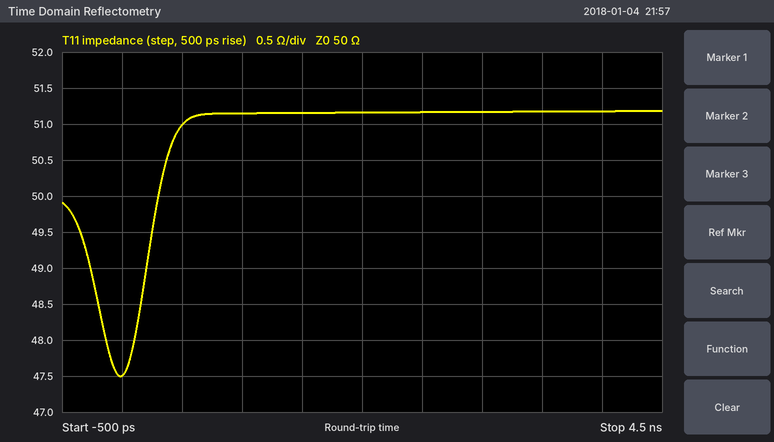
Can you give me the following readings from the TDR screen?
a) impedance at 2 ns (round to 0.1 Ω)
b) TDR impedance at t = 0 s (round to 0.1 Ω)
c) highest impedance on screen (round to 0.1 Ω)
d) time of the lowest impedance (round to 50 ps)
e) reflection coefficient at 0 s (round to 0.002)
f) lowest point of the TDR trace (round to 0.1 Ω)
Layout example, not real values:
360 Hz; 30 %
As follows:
51.2 Ω; 47.5 Ω; 51.2 Ω; 0 ps; -0.026; 47.5 Ω
